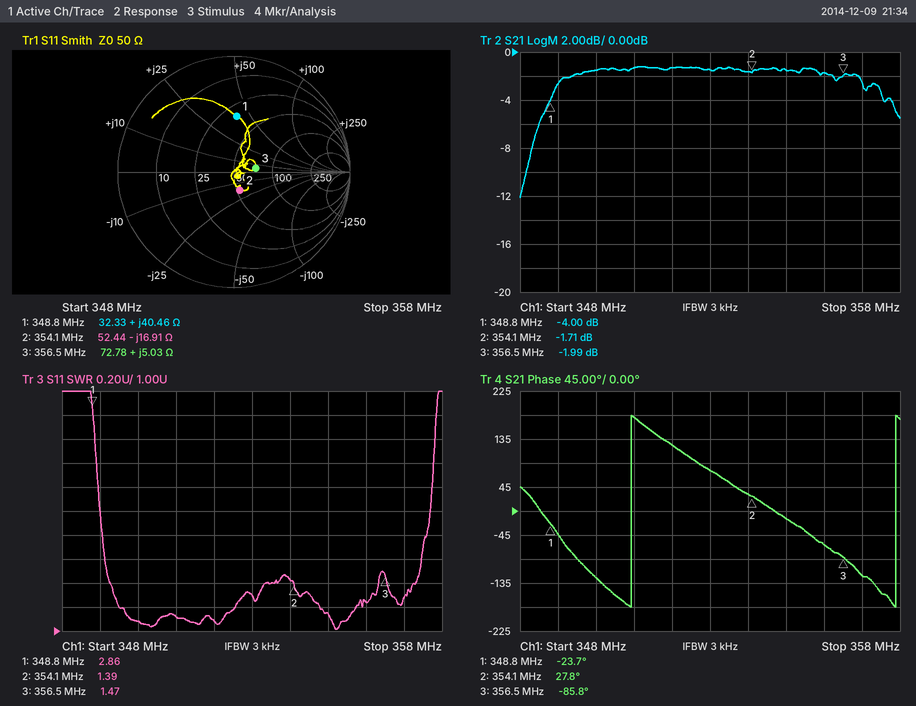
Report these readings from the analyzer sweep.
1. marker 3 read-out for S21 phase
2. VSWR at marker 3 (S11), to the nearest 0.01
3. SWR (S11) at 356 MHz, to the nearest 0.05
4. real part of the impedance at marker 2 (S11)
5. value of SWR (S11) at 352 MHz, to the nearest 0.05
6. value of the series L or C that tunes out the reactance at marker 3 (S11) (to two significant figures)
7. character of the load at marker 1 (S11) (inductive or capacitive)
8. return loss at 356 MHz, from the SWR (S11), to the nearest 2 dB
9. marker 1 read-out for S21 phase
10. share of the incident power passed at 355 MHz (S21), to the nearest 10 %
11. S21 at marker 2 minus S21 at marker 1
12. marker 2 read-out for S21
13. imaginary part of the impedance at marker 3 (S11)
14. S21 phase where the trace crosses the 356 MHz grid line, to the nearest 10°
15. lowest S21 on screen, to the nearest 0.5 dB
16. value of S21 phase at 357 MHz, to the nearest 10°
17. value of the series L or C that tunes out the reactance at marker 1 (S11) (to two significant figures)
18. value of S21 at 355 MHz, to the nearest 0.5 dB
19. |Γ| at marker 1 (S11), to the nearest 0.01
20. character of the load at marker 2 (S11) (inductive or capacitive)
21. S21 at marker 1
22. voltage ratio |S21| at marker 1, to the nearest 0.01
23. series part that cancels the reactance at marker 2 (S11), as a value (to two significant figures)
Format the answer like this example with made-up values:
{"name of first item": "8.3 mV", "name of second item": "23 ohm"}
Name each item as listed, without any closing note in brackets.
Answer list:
{"marker 3 read-out for S21 phase": "-85.8°", "VSWR at marker 3 (S11), to the nearest 0.01": "1.47", "SWR (S11) at 356 MHz, to the nearest 0.05": "1.25", "real part of the impedance at marker 2": "52.44 Ω", "value of SWR (S11) at 352 MHz, to the nearest 0.05": "1.10", "value of the series L or C that tunes out the reactance at marker 3 (S11)": "89 pF", "character of the load at marker 1 (S11)": "inductive", "return loss at 356 MHz, from the SWR (S11), to the nearest 2 dB": "20 dB", "marker 1 read-out for S21 phase": "-23.7°", "share of the incident power passed at 355 MHz (S21), to the nearest 10 %": "70 %", "S21 at marker 2 minus S21 at marker 1": "2.29 dB", "marker 2 read-out for S21": "-1.71 dB", "imaginary part of the impedance at marker 3": "+5.03 Ω", "S21 phase where the trace crosses the 356 MHz grid line, to the nearest 10°": "-60°", "lowest S21 on screen, to the nearest 0.5 dB": "-12.0 dB", "value of S21 phase at 357 MHz, to the nearest 10°": "-120°", "value of the series L or C that tunes out the reactance at marker 1 (S11)": "11 pF", "value of S21 at 355 MHz, to the nearest 0.5 dB": "-1.5 dB", "|Γ| at marker 1 (S11), to the nearest 0.01": "0.48", "character of the load at marker 2 (S11)": "capacitive", "S21 at marker 1": "-4.00 dB", "voltage ratio |S21| at marker 1, to the nearest 0.01": "0.63", "series part that cancels the reactance at marker 2 (S11), as a value": "7.6 nH"}
